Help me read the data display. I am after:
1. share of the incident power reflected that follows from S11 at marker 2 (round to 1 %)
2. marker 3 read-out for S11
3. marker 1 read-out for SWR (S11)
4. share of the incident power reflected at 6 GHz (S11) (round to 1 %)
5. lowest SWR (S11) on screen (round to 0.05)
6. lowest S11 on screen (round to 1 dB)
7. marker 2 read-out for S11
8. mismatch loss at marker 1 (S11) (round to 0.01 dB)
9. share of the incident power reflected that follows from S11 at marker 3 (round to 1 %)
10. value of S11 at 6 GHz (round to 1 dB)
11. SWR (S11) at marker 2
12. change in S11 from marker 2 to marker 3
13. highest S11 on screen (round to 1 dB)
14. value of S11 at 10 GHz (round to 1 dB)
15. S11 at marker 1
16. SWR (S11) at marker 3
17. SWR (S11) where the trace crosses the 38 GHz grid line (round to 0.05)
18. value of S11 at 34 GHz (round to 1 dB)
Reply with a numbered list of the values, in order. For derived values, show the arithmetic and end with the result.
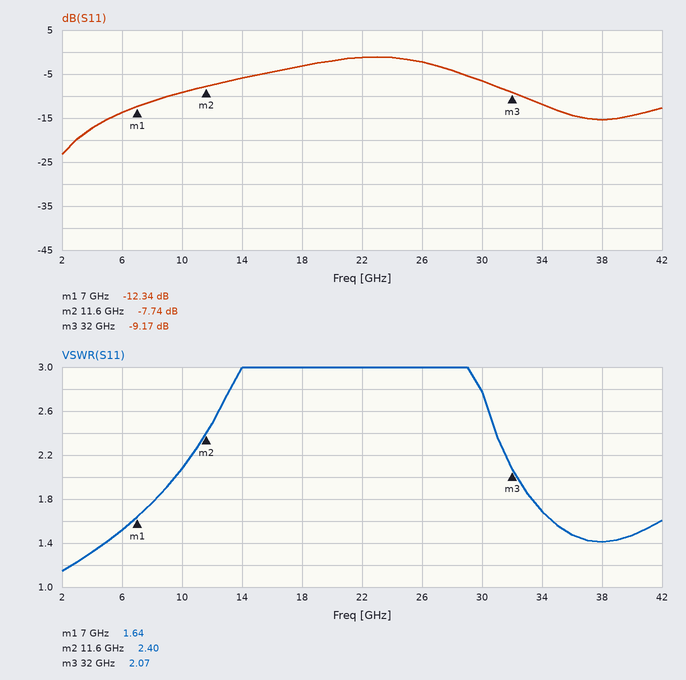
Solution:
1. 10^(-7.74/10) ≈ 17 %
2. -9.17 dB
3. 1.64
4. 10^(-14/10) ≈ 4 %
5. 1.15
6. -23 dB
7. -7.74 dB
8. −10 log10(1 − 10^(-12.34/10)) ≈ 0.26 dB
9. 10^(-9.17/10) ≈ 12 %
10. -14 dB
11. 2.40
12. -9.17 − (-7.74) = -1.43 dB
13. -1 dB
14. -9 dB
15. -12.34 dB
16. 2.07
17. 1.40
18. -12 dB
